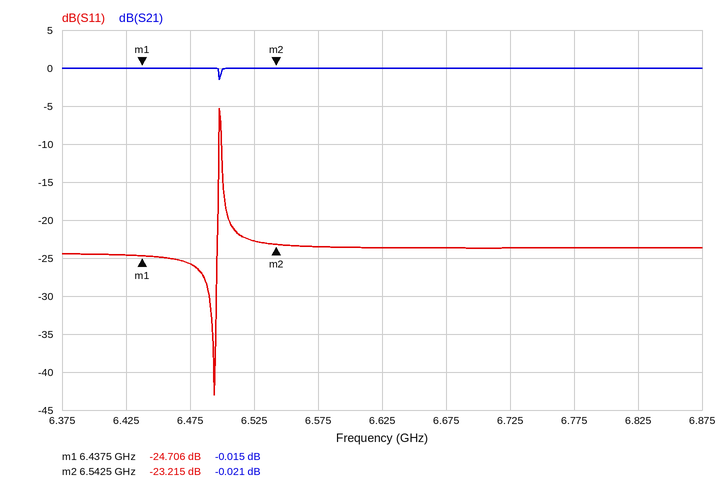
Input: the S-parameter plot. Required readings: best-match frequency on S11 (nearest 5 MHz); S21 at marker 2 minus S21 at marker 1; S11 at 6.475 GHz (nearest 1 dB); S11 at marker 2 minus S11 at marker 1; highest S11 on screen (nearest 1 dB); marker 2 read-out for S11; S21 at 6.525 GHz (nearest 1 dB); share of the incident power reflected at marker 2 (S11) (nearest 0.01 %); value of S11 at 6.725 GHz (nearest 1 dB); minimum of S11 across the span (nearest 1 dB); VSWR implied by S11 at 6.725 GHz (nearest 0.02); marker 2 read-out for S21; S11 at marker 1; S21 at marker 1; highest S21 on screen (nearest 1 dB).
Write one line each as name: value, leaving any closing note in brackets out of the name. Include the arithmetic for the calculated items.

best-match frequency on S11: 6.495 GHz
S21 at marker 2 minus S21 at marker 1: -0.021 − (-0.015) = -0.006 dB
S11 at 6.475 GHz: -26 dB
S11 at marker 2 minus S11 at marker 1: -23.215 − (-24.706) = 1.491 dB
highest S11 on screen: -5 dB
marker 2 read-out for S11: -23.215 dB
S21 at 6.525 GHz: 0 dB
share of the incident power reflected at marker 2 (S11): 10^(-23.215/10) ≈ 0.48 %
value of S11 at 6.725 GHz: -24 dB
minimum of S11 across the span: -43 dB
VSWR implied by S11 at 6.725 GHz: |Γ| = 10^(-24/20) = 0.0631; VSWR = (1 + 0.0631)/(1 − 0.0631) ≈ 1.13, so 1.14 to the nearest 0.02
marker 2 read-out for S21: -0.021 dB
S11 at marker 1: -24.706 dB
S21 at marker 1: -0.015 dB
highest S21 on screen: 0 dB
